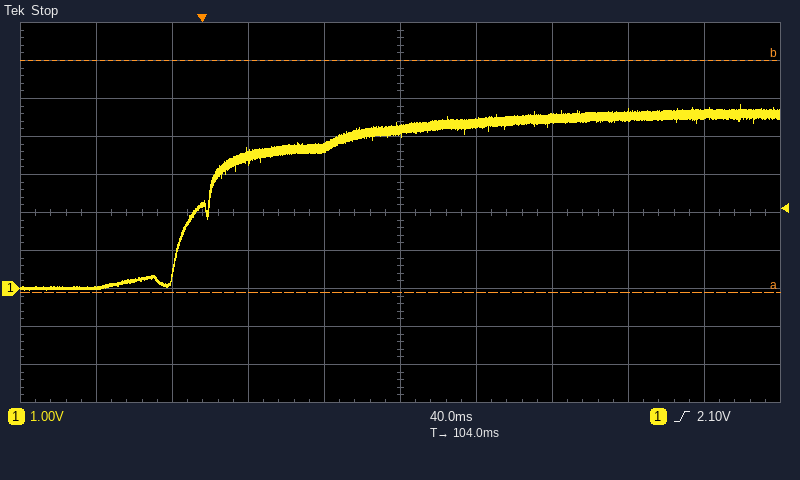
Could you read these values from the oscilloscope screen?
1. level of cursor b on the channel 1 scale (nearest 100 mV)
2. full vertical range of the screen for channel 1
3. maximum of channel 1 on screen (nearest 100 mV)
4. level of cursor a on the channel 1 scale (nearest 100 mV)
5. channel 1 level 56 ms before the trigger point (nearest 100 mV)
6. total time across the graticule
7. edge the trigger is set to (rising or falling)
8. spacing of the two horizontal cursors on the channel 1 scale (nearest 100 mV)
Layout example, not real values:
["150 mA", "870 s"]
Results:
["6.0 V", "10 V", "4.8 V", "-100 mV", "0.0 V", "400 ms", "rising", "6.1 V"]
